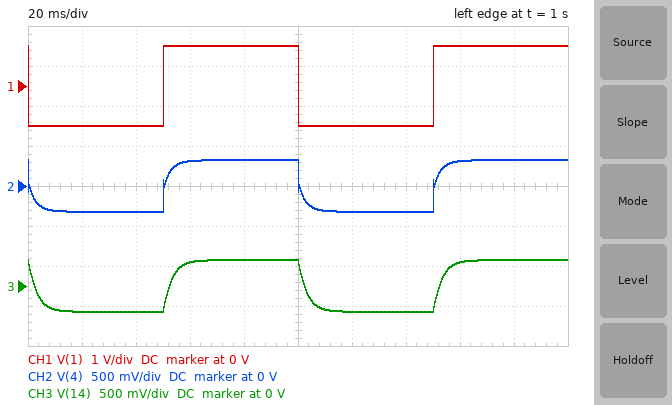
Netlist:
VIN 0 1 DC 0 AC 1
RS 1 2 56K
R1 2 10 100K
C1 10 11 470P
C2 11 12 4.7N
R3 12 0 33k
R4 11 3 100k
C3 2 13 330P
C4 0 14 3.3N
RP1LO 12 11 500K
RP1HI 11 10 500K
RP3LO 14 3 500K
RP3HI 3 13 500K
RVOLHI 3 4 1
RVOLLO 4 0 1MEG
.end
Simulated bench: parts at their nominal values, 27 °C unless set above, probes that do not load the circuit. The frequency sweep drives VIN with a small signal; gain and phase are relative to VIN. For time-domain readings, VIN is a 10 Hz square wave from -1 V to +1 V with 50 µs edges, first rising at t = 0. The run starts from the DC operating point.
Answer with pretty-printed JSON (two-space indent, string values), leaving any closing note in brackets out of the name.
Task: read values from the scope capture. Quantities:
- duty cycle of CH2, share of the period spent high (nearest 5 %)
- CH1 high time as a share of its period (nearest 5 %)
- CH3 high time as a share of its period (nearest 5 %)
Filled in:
{
  "duty cycle of CH2, share of the period spent high": "50 %",
  "CH1 high time as a share of its period": "50 %",
  "CH3 high time as a share of its period": "50 %"
}
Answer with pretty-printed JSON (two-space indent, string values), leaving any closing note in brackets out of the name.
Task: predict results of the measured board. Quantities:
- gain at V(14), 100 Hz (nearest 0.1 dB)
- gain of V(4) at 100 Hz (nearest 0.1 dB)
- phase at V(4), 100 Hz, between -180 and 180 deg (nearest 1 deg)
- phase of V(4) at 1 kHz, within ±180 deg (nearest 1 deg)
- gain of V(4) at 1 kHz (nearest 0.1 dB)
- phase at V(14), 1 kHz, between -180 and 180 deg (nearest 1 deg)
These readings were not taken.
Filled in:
{
  "gain at V(14), 100 Hz": "-17.2 dB",
  "gain of V(4) at 100 Hz": "-14.0 dB",
  "phase at V(4), 100 Hz, between -180 and 180 deg": "157 deg",
  "phase of V(4) at 1 kHz, within ±180 deg": "-169 deg",
  "gain of V(4) at 1 kHz": "-15.5 dB",
  "phase at V(14), 1 kHz, between -180 and 180 deg": "106 deg"
}
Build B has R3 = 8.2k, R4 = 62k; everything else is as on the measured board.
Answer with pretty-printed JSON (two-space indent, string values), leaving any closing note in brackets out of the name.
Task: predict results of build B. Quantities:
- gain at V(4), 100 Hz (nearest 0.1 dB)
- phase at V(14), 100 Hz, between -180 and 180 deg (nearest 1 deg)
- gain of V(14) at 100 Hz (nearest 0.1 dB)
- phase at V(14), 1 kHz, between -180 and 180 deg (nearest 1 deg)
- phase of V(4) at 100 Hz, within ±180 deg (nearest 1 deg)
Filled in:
{
  "gain at V(4), 100 Hz": "-13.7 dB",
  "phase at V(14), 100 Hz, between -180 and 180 deg": "109 deg",
  "gain of V(14) at 100 Hz": "-16.9 dB",
  "phase at V(14), 1 kHz, between -180 and 180 deg": "89 deg",
  "phase of V(4) at 100 Hz, within ±180 deg": "155 deg"
}
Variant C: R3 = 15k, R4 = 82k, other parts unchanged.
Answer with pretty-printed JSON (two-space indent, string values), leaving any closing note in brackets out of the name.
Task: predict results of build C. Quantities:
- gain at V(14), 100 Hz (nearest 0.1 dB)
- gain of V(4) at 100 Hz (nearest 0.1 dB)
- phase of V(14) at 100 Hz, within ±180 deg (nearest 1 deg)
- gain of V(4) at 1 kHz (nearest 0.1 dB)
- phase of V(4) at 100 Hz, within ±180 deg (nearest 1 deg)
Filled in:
{
  "gain at V(14), 100 Hz": "-17.1 dB",
  "gain of V(4) at 100 Hz": "-13.9 dB",
  "phase of V(14) at 100 Hz, within ±180 deg": "109 deg",
  "gain of V(4) at 1 kHz": "-17.2 dB",
  "phase of V(4) at 100 Hz, within ±180 deg": "155 deg"
}
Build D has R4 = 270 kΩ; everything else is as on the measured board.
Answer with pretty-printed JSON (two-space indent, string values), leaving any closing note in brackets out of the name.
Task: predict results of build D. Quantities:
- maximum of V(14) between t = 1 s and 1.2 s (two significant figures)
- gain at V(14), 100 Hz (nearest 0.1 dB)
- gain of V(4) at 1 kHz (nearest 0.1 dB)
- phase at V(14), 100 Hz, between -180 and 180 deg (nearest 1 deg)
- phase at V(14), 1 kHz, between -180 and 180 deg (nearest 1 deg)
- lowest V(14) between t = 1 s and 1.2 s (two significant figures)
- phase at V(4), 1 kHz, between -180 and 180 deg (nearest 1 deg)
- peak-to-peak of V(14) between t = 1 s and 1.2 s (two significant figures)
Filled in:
{
  "maximum of V(14) between t = 1 s and 1.2 s": "290 mV",
  "gain at V(14), 100 Hz": "-19.0 dB",
  "gain of V(4) at 1 kHz": "-13.8 dB",
  "phase at V(14), 100 Hz, between -180 and 180 deg": "111 deg",
  "phase at V(14), 1 kHz, between -180 and 180 deg": "113 deg",
  "lowest V(14) between t = 1 s and 1.2 s": "-290 mV",
  "phase at V(4), 1 kHz, between -180 and 180 deg": "-163 deg",
  "peak-to-peak of V(14) between t = 1 s and 1.2 s": "570 mV"
}
